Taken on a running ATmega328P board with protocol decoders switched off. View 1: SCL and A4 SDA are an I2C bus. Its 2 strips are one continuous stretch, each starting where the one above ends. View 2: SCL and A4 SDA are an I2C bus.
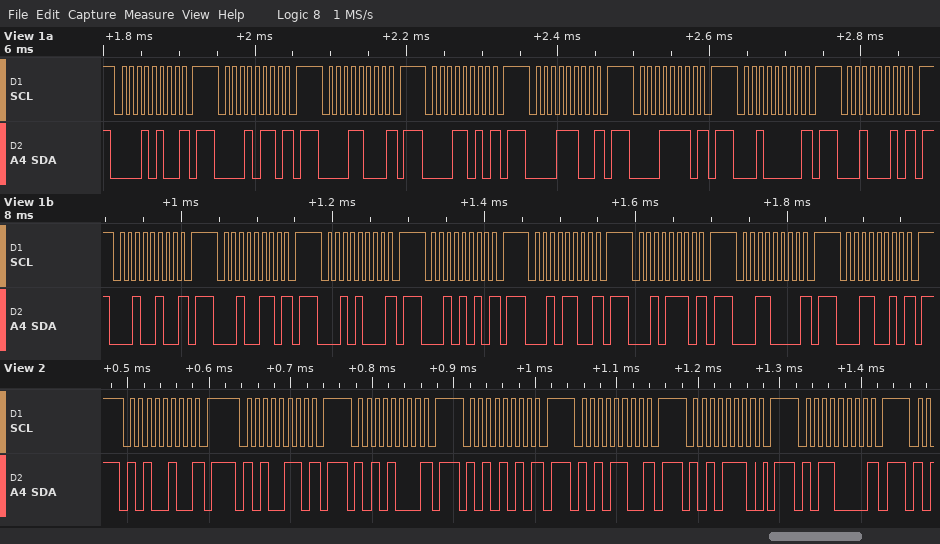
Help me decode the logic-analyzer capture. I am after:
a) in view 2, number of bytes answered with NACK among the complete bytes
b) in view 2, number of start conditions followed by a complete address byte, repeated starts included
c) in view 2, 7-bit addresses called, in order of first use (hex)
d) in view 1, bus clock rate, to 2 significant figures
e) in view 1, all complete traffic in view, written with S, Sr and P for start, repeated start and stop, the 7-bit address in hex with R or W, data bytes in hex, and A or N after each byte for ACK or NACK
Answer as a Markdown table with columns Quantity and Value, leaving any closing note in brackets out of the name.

| Quantity | Value |
|---|---|
| in view 2, number of bytes answered with NACK among the complete bytes | 6 |
| in view 2, number of start conditions followed by a complete address byte, repeated starts included | 7 |
| in view 2, 7-bit addresses called, in order of first use | 0x52 0x53 0x54 0x55 0x56 0x57 0x58 |
| in view 1, bus clock rate, to 2 significant figures | 100 kHz |
| in view 1, all complete traffic in view, written with S, Sr and P for start, repeated start and stop, the 7-bit address in hex with R or W, data bytes in hex, and A or N after each byte for ACK or NACK | S 0AW N P S 0BW N P S 0CW N P S 0DW N P S 0EW N P S 0FW N P S 10W N P S 11W N P S 12W N P S 13W N P S 14W N P S 15W N P S 16W N P S 17W N P S 18W N P S 19W N P |
